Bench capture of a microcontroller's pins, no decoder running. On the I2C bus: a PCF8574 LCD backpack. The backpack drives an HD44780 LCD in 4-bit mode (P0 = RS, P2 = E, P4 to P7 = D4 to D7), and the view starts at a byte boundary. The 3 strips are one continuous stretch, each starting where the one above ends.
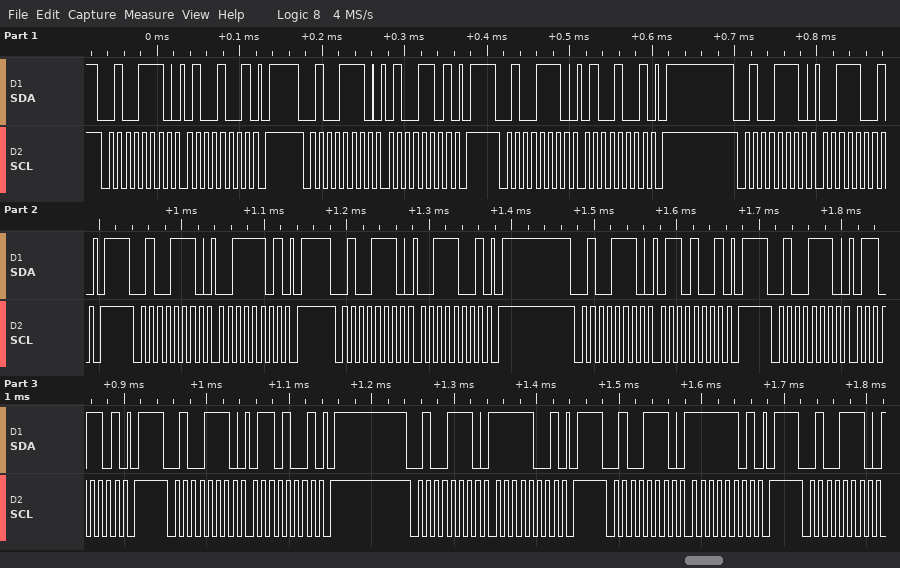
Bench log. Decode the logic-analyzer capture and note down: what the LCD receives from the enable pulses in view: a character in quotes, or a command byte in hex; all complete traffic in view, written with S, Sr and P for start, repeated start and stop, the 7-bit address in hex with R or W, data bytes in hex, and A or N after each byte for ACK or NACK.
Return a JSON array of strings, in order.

["'C'", "S 27W A 49 A P S 27W A 4D A P S 27W A 49 A P S 27W A 39 A P S 27W A 3D A P S 27W A 39 A P S 27W A 69 A P S 27W A 6D A P S 27W A 69 A P S 27W A F9 A P S 27W A FD A P S 27W A"]
